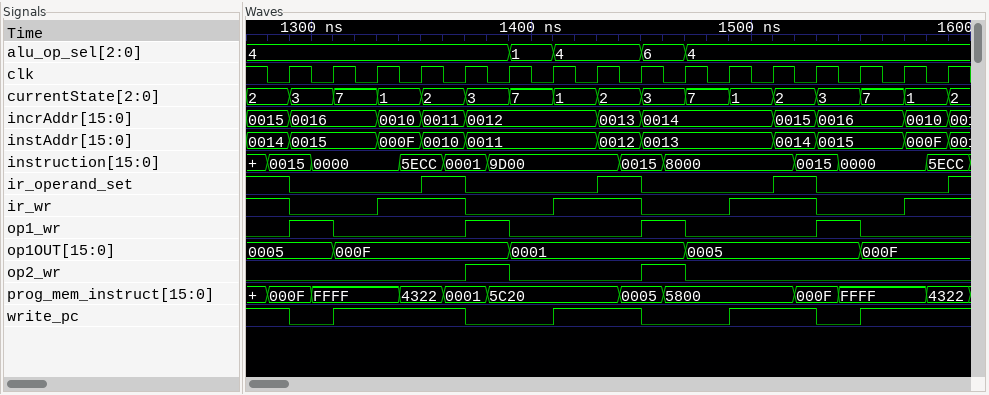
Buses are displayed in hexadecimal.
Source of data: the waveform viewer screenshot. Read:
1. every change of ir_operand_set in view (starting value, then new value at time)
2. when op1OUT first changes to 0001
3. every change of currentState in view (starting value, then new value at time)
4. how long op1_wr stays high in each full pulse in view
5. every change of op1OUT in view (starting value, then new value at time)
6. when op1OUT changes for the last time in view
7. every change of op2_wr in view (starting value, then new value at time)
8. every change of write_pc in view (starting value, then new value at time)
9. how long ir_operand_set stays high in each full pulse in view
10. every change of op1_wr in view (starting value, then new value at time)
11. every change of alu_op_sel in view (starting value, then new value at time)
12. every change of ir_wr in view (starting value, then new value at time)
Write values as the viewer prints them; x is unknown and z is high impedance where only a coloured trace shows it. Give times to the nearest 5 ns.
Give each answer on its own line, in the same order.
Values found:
1, 0 at 1290 ns, 1 at 1350 ns, 0 at 1370 ns, 1 at 1430 ns, 0 at 1450 ns, 1 at 1510 ns, 0 at 1530 ns, 1 at 1590 ns
1390 ns
2, 3 at 1290 ns, 7 at 1310 ns, 1 at 1330 ns, 2 at 1350 ns, 3 at 1370 ns, 7 at 1390 ns, 1 at 1410 ns, 2 at 1430 ns, 3 at 1450 ns, 7 at 1470 ns, 1 at 1490 ns, 2 at 1510 ns, 3 at 1530 ns, 7 at 1550 ns, 1 at 1570 ns, 2 at 1590 ns
20 ns, 20 ns, 20 ns, 20 ns
0005, 000F at 1310 ns, 0001 at 1390 ns, 0005 at 1470 ns, 000F at 1550 ns
1550 ns
0, 1 at 1370 ns, 0 at 1390 ns, 1 at 1450 ns, 0 at 1470 ns
1, 0 at 1290 ns, 1 at 1310 ns, 0 at 1370 ns, 1 at 1410 ns, 0 at 1450 ns, 1 at 1490 ns, 0 at 1530 ns, 1 at 1550 ns
20 ns, 20 ns, 20 ns
0, 1 at 1290 ns, 0 at 1310 ns, 1 at 1370 ns, 0 at 1390 ns, 1 at 1450 ns, 0 at 1470 ns, 1 at 1530 ns, 0 at 1550 ns
4, 1 at 1390 ns, 4 at 1410 ns, 6 at 1450 ns, 4 at 1470 ns
1, 0 at 1290 ns, 1 at 1330 ns, 0 at 1370 ns, 1 at 1410 ns, 0 at 1450 ns, 1 at 1490 ns, 0 at 1530 ns, 1 at 1570 ns
